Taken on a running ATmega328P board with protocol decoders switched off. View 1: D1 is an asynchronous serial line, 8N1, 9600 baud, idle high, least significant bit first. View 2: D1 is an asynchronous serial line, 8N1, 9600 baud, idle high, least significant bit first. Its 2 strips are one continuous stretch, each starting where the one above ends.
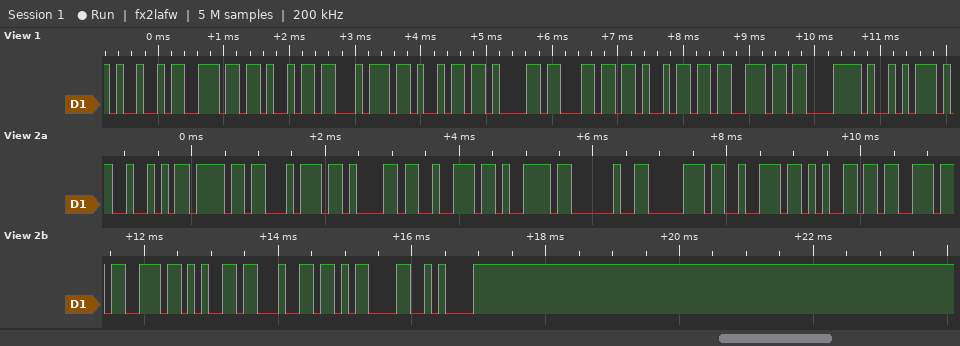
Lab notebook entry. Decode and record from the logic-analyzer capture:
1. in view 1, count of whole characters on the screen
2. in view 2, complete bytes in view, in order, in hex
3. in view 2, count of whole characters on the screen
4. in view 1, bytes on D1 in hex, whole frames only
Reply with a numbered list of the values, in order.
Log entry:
1. 11
2. 0x52 0x6F 0x74 0x61 0x72 0x79 0x20 0x70 0x72 0x65 0x73 0x73 0x65 0x64 0x0D 0x0A
3. 16
4. 0x49 0x6E 0x69 0x74 0x69 0x61 0x6C 0x69 0x73 0xC3 0xA9
